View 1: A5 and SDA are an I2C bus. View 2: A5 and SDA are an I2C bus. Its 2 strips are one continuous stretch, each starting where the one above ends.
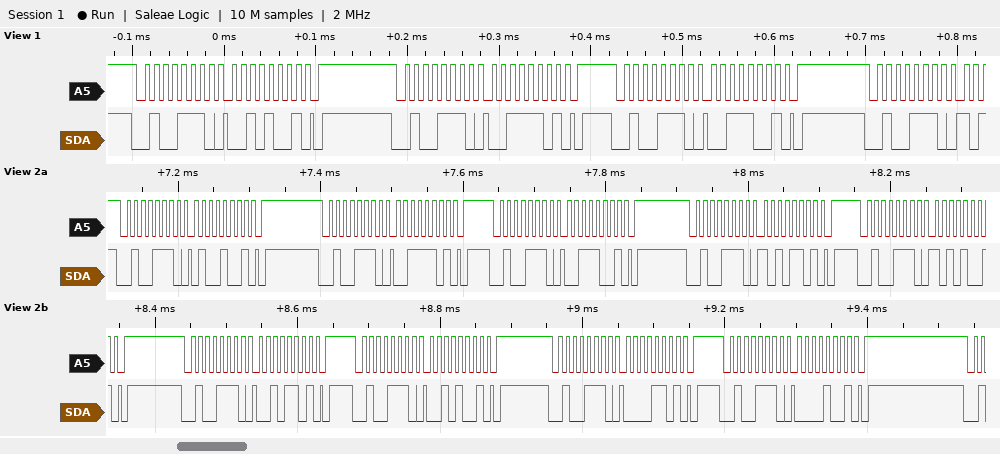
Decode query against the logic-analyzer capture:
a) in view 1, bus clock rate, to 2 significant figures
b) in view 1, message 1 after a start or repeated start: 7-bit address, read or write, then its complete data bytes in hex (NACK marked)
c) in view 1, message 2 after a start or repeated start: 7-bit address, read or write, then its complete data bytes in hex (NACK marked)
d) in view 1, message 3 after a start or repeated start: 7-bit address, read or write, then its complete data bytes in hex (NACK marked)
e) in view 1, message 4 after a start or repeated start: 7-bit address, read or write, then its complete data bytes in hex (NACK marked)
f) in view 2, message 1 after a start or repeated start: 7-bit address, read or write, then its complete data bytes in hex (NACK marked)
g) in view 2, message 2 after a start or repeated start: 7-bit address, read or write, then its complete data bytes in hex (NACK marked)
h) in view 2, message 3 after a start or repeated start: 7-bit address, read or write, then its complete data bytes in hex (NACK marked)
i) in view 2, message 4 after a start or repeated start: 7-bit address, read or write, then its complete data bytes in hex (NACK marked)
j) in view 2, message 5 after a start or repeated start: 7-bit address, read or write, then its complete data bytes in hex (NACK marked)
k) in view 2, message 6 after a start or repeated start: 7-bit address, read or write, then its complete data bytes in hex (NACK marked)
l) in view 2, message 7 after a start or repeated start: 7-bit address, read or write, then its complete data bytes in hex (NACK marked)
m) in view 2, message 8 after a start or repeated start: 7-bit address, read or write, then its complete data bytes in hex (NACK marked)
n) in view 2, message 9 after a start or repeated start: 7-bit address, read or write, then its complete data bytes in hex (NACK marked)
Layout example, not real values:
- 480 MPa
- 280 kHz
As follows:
- 100 kHz
- 0x27 write: 29
- 0x27 write: 3D
- 0x27 write: 39
- 0x27 write
- 0x27 write: 49
- 0x27 write: 3D
- 0x27 write: 39
- 0x27 write: AD
- 0x27 write: A9
- 0x27 write: 2D
- 0x27 write: 29
- 0x27 write: 0D
- 0x27 write: 09
